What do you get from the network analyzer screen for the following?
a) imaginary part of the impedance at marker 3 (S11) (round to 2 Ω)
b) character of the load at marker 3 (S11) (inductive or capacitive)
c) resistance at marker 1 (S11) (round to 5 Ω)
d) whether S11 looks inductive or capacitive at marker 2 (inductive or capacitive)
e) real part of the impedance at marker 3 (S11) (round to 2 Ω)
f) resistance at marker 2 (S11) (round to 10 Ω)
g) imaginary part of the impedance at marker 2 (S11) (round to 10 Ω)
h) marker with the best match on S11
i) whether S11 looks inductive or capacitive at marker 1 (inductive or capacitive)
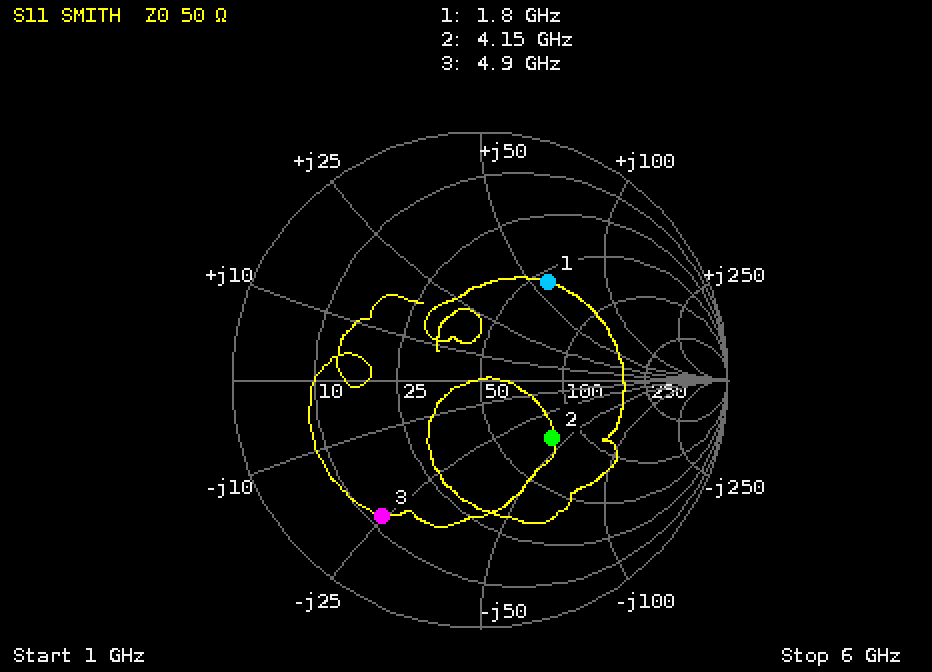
-24 Ω
capacitive
55 Ω
capacitive
12 Ω
80 Ω
-40 Ω
marker 2
inductive
